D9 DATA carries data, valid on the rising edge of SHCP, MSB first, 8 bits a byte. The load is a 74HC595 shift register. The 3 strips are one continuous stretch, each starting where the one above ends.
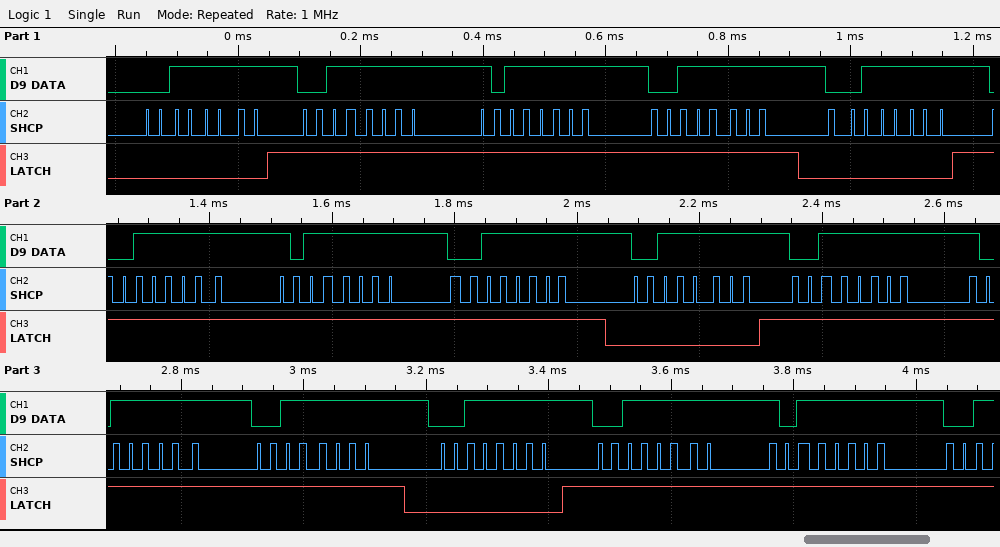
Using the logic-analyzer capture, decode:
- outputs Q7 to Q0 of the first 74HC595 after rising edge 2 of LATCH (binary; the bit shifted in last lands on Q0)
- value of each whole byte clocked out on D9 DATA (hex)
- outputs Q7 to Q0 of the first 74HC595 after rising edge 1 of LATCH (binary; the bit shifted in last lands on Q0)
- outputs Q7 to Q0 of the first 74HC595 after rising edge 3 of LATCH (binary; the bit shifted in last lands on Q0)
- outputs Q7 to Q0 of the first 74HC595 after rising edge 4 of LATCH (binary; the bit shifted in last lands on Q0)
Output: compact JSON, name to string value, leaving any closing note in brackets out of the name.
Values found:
{"outputs Q7 to Q0 of the first 74HC595 after rising edge 2 of LATCH": "00111111", "value of each whole byte clocked out on D9 DATA": "0x3F 0x3F 0xBF 0x3F 0x3F 0x3F 0xBF 0x3F 0x3F 0x3F 0xBF 0x3F 0x3F 0x3F 0xBF", "outputs Q7 to Q0 of the first 74HC595 after rising edge 1 of LATCH": "00111111", "outputs Q7 to Q0 of the first 74HC595 after rising edge 3 of LATCH": "00111111", "outputs Q7 to Q0 of the first 74HC595 after rising edge 4 of LATCH": "00111111"}
